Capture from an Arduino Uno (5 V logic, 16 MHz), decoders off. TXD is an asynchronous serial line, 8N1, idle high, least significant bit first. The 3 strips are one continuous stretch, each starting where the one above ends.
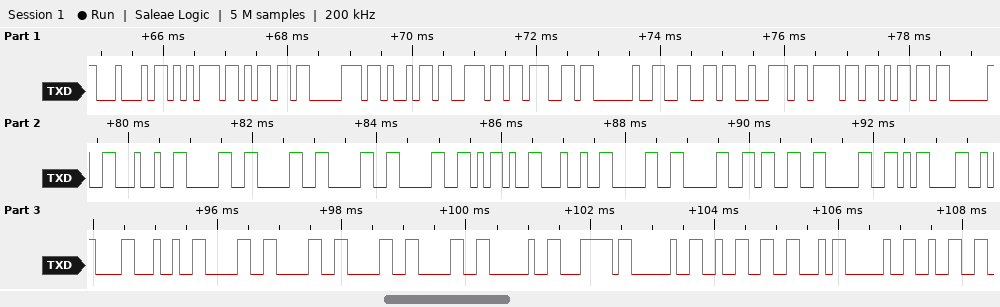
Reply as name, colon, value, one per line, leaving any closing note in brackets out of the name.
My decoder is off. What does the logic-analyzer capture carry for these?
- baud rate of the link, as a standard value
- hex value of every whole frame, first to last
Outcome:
baud rate of the link, as a standard value: 9600 baud
hex value of every whole frame, first to last: 44 75 6D 70 69 6E 67 20 66 72 6F 6D 20 24 30 30 30 30 2D 24 30 30 33 30 0D 0A 24 30 30 30 30 20 7C 20 32 46 20 32
